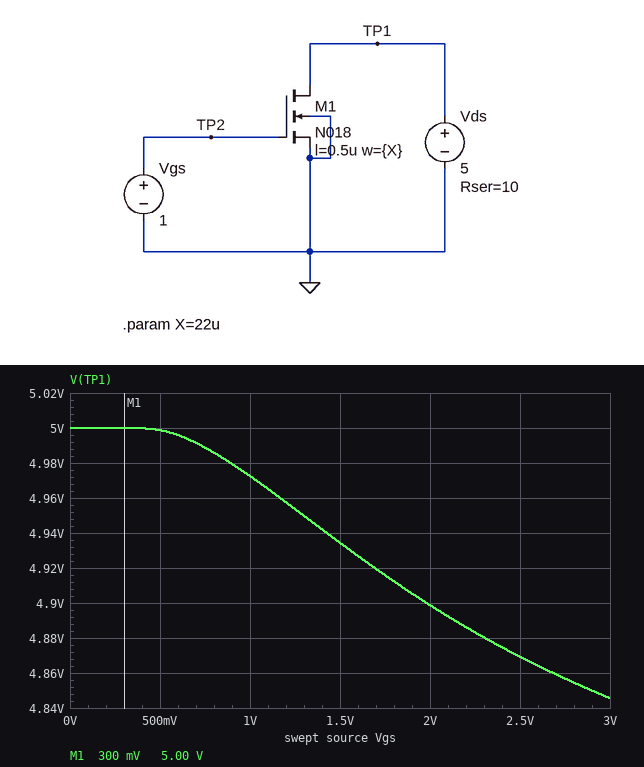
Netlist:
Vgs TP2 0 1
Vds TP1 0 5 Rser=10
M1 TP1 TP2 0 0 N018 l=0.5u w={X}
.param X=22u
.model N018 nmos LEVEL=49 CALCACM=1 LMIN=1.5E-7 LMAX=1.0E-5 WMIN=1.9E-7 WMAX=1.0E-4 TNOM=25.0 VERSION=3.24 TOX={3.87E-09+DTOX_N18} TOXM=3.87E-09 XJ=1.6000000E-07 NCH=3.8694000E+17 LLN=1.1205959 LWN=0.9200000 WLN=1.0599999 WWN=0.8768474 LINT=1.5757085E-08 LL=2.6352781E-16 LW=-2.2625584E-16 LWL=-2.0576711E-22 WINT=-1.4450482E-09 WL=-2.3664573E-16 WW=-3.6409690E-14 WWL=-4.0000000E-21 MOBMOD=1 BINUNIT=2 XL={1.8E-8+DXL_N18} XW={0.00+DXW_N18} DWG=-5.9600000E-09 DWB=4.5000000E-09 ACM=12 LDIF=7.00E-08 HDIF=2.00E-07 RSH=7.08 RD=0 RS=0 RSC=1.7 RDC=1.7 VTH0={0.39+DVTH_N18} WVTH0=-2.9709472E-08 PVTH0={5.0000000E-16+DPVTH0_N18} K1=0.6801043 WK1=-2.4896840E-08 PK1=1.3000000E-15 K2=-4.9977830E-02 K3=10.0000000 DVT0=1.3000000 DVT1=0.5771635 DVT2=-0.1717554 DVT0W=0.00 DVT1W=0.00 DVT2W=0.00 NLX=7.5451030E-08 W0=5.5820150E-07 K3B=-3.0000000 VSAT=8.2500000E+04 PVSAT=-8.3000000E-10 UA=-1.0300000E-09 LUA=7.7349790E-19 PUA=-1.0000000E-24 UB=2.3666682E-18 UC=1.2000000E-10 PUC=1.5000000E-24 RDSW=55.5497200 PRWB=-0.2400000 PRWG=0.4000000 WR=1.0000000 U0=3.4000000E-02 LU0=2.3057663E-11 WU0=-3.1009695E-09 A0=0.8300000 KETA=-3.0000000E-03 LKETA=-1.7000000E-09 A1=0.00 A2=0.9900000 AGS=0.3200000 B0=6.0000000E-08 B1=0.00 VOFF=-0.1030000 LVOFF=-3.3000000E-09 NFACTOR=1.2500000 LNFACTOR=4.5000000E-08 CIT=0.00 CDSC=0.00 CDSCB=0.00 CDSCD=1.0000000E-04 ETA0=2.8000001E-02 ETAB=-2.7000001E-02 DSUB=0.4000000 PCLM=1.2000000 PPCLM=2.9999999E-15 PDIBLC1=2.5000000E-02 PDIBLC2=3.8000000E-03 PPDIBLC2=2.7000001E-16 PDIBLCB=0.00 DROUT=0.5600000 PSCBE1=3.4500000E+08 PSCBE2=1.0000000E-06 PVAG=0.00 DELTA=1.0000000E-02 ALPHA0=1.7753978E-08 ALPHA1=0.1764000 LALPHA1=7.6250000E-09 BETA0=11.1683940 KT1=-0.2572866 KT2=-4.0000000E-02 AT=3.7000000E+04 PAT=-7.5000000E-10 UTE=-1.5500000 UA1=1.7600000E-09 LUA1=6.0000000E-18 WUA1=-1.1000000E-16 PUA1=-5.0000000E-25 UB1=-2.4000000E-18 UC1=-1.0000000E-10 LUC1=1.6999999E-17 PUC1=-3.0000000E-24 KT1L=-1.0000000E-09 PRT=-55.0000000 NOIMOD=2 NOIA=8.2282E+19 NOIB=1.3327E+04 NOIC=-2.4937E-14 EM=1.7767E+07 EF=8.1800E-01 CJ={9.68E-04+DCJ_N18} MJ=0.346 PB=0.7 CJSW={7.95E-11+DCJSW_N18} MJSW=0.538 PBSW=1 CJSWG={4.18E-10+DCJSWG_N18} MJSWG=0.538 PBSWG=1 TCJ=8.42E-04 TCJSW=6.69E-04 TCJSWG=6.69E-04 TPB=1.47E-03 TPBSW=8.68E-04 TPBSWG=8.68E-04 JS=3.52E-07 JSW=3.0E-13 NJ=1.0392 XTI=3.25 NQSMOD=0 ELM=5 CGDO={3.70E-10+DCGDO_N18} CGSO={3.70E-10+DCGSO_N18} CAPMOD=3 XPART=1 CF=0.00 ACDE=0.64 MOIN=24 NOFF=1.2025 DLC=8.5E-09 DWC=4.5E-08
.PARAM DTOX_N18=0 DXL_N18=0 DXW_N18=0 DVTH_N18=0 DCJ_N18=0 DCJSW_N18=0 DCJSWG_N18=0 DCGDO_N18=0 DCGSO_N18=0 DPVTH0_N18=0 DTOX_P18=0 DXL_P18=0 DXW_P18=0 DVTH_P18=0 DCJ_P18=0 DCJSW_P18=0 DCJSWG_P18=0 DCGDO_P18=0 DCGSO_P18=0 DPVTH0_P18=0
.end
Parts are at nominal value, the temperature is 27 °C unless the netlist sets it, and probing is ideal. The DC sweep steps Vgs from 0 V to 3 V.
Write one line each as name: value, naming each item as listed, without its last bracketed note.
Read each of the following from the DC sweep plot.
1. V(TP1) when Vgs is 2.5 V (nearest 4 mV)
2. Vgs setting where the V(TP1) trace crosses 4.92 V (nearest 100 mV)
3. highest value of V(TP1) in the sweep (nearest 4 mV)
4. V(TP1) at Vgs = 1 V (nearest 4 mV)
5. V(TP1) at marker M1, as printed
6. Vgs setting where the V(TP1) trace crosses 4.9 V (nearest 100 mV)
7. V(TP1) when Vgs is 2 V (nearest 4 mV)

V(TP1) when Vgs is 2.5 V: 4.868 V
Vgs setting where the V(TP1) trace crosses 4.92 V: 1.7 V
highest value of V(TP1) in the sweep: 5.000 V
V(TP1) at Vgs = 1 V: 4.972 V
V(TP1) at marker M1, as printed: 5.00 V
Vgs setting where the V(TP1) trace crosses 4.9 V: 2.0 V
V(TP1) when Vgs is 2 V: 4.900 V
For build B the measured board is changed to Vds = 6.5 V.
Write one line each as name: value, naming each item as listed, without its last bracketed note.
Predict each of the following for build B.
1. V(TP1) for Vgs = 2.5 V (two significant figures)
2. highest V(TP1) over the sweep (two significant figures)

V(TP1) for Vgs = 2.5 V: 6.3 V
highest V(TP1) over the sweep: 6.5 V
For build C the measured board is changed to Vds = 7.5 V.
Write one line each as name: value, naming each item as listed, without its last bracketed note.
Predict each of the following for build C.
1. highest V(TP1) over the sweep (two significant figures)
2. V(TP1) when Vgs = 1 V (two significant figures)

highest V(TP1) over the sweep: 7.5 V
V(TP1) when Vgs = 1 V: 7.4 V
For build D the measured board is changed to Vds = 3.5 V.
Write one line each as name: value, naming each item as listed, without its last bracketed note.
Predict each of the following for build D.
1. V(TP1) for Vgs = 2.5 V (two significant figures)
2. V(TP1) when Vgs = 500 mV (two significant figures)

V(TP1) for Vgs = 2.5 V: 3.4 V
V(TP1) when Vgs = 500 mV: 3.5 V
